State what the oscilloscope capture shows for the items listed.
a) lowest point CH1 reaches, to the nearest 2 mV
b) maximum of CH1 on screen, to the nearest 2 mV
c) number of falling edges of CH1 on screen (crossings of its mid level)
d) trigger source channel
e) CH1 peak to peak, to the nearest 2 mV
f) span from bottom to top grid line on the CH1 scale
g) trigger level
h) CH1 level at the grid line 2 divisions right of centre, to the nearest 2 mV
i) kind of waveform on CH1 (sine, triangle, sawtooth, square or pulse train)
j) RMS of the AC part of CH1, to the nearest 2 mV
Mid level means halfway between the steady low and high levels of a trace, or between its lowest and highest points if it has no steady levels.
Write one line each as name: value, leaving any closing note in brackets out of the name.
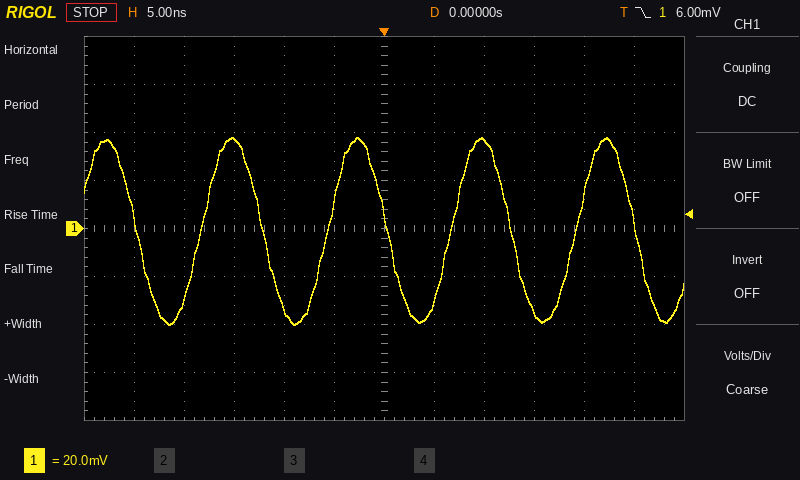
lowest point CH1 reaches, to the nearest 2 mV: -40 mV
maximum of CH1 on screen, to the nearest 2 mV: 38 mV
number of falling edges of CH1 on screen: 5
trigger source channel: CH1
CH1 peak to peak, to the nearest 2 mV: 78 mV
span from bottom to top grid line on the CH1 scale: 160 mV
trigger level: 6.00 mV
CH1 level at the grid line 2 divisions right of centre, to the nearest 2 mV: 36 mV
kind of waveform on CH1: sine
RMS of the AC part of CH1, to the nearest 2 mV: 28 mV
